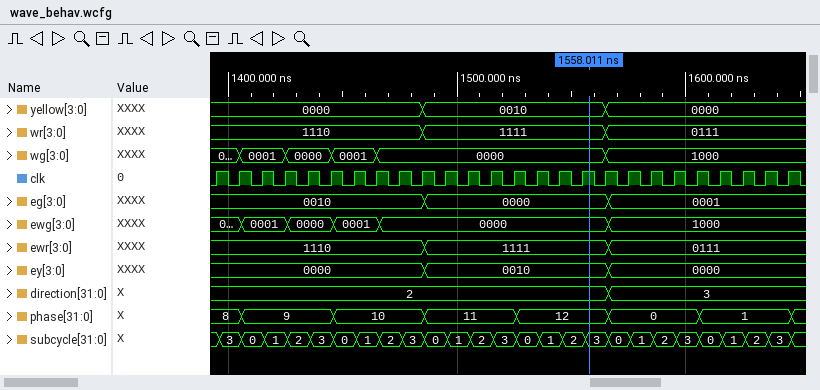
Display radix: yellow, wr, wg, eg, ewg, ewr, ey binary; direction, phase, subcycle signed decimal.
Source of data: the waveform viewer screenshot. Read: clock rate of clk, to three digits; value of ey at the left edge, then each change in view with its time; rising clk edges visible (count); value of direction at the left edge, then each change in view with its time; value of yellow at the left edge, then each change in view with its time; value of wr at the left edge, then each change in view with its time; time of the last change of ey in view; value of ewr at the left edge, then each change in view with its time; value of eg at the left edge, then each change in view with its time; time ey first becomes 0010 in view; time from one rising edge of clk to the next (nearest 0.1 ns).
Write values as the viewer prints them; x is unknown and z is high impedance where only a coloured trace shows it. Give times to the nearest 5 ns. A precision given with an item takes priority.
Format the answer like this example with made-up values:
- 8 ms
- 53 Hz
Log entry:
- 100 MHz
- 0000, 0010 at 1485 ns, 0000 at 1565 ns
- 26
- 2, 3 at 1565 ns
- 0000, 0010 at 1485 ns, 0000 at 1565 ns
- 1110, 1111 at 1485 ns, 0111 at 1565 ns
- 1565 ns
- 1110, 1111 at 1485 ns, 0111 at 1565 ns
- 0010, 0000 at 1485 ns, 0001 at 1565 ns
- 1485 ns
- 10 ns
